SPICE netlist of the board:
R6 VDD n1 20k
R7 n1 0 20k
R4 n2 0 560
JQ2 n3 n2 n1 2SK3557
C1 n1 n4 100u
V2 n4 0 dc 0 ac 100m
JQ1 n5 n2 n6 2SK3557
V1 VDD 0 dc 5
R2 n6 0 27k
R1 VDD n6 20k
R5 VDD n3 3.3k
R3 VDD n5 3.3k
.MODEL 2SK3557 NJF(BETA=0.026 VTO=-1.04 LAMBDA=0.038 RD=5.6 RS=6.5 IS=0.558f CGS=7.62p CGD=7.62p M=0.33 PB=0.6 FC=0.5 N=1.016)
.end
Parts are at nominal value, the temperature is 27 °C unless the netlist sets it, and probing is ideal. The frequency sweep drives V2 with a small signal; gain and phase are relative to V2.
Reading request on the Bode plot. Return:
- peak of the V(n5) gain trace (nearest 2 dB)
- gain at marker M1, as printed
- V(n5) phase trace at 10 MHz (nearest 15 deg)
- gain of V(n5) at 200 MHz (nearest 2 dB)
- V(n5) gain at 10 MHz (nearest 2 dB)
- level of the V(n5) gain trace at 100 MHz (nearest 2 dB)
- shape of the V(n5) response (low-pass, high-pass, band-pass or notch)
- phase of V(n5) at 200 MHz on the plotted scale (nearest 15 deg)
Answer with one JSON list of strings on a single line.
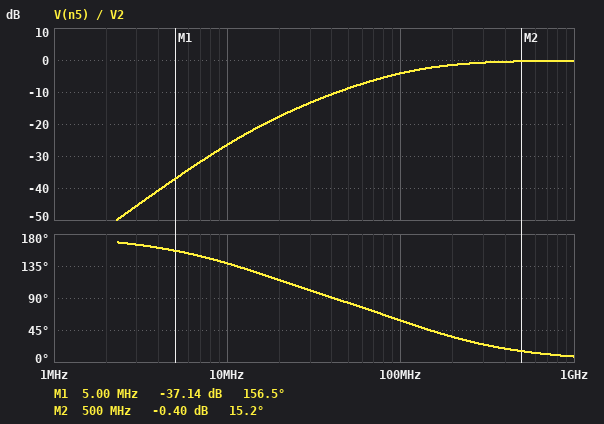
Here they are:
["0 dB", "-37.14 dB", "135 deg", "-2 dB", "-26 dB", "-4 dB", "high-pass", "30 deg"]
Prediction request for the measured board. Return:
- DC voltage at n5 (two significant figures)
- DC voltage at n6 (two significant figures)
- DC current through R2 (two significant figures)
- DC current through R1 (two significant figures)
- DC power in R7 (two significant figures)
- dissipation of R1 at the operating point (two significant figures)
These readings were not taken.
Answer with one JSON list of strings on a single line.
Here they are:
["5.0 V", "2.9 V", "110 µA", "110 µA", "310 µW", "230 µW"]
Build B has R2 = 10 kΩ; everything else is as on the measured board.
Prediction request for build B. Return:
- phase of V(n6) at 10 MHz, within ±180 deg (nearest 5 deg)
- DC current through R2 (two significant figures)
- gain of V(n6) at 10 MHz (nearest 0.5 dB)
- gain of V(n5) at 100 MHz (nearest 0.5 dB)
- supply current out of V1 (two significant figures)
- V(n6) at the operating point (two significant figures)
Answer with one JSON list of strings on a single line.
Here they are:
["105 deg", "170 µA", "-21.5 dB", "-4.5 dB", "290 µA", "1.7 V"]
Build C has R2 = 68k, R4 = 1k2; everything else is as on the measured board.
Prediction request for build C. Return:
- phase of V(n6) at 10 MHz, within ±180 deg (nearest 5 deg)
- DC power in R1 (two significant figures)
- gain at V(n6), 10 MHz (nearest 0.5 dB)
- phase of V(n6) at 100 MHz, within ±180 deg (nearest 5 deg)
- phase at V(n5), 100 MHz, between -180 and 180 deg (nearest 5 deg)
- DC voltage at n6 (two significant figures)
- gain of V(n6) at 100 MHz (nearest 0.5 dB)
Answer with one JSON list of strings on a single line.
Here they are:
["85 deg", "65 µW", "-15.0 dB", "35 deg", "45 deg", "3.9 V", "-2.0 dB"]
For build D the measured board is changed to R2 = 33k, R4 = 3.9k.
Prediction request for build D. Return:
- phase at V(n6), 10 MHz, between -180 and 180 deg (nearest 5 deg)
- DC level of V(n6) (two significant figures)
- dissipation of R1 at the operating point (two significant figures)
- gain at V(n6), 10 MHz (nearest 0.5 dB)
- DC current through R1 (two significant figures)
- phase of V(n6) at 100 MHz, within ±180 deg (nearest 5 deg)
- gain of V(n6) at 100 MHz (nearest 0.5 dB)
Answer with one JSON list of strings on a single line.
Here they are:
["65 deg", "3.1 V", "180 µW", "-10.5 dB", "94 µA", "25 deg", "-1.0 dB"]
